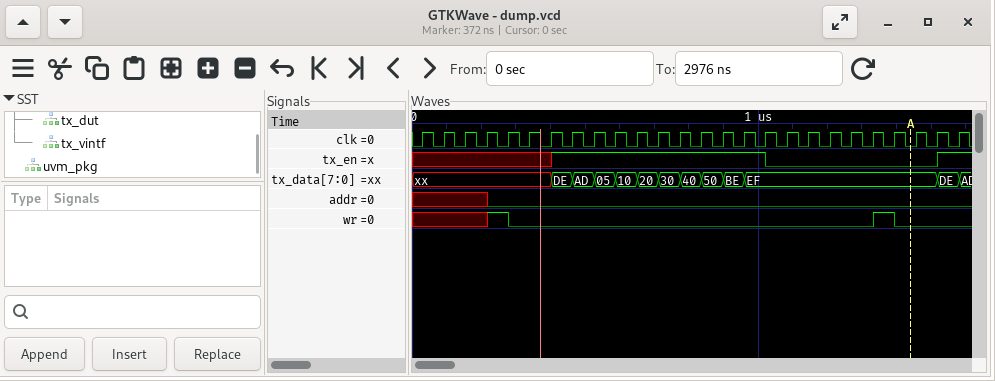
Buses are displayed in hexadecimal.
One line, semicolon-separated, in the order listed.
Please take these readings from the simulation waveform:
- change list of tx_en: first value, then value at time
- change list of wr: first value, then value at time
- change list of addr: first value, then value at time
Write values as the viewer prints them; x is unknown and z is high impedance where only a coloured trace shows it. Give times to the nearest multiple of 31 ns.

x, 1 at 403 ns, 0 at 1023 ns, 1 at 1519 ns; x, 1 at 217 ns, 0 at 279 ns, 1 at 1333 ns, 0 at 1395 ns; x, 0 at 217 ns
